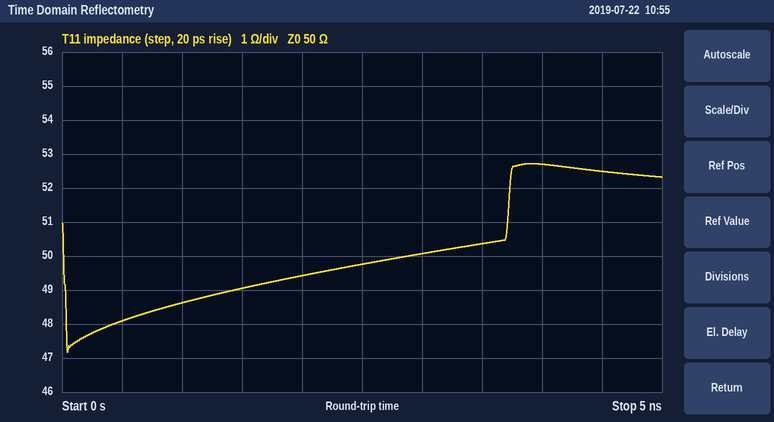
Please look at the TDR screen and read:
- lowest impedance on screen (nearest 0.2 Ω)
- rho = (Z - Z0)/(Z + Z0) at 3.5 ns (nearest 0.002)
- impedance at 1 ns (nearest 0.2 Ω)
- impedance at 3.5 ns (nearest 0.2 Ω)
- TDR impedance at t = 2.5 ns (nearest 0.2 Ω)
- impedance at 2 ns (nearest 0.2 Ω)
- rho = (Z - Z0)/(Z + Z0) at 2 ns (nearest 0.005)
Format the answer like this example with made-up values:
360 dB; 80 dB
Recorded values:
47.2 Ω; +0.004; 48.6 Ω; 50.4 Ω; 49.8 Ω; 49.4 Ω; -0.005
